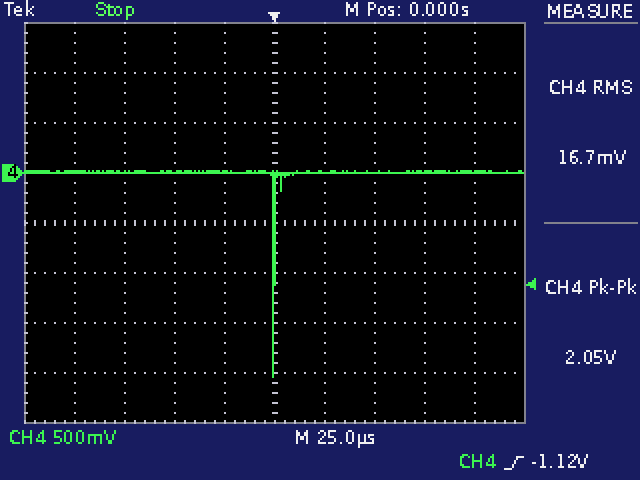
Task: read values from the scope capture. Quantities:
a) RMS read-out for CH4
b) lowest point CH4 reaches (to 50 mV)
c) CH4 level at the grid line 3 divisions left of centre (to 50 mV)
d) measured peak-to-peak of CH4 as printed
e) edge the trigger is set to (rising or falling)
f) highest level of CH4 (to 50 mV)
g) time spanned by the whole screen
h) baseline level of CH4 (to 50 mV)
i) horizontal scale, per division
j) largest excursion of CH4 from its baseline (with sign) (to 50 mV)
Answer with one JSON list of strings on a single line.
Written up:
["16.7 mV", "-2.05 V", "0 mV", "2.05 V", "rising", "0 mV", "250 µs", "0 mV", "25 µs", "-2.05 V"]
